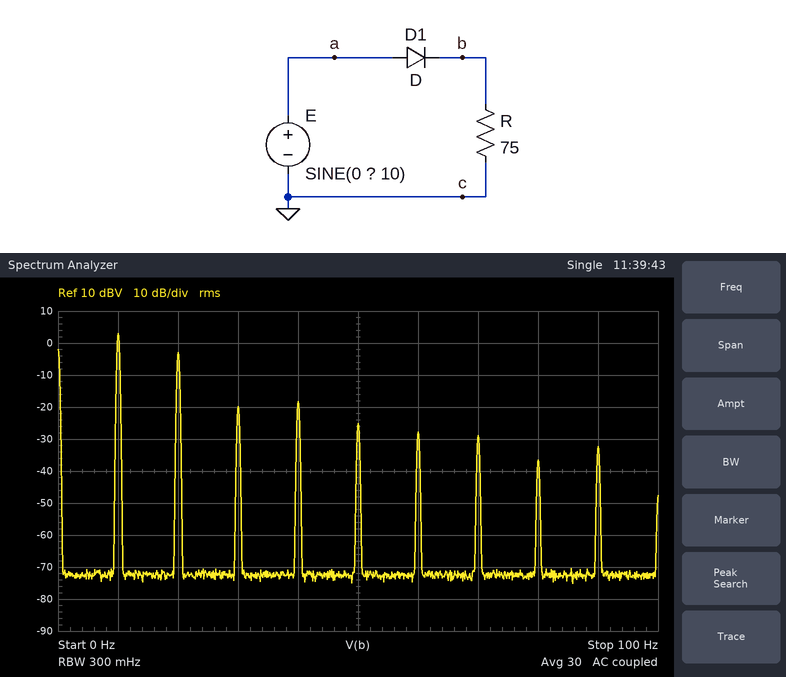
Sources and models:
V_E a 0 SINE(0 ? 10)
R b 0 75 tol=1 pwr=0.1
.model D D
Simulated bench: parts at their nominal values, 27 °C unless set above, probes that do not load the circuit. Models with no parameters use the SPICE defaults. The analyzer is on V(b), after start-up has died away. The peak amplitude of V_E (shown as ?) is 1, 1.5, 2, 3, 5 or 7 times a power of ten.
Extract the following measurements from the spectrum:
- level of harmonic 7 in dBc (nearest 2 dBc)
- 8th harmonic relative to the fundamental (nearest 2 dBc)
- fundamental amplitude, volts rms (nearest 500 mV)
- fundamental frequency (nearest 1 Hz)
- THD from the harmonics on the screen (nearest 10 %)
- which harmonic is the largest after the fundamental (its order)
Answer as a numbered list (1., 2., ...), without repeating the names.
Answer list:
1. -32 dBc
2. -40 dBc
3. 1.5 V
4. 10 Hz
5. 50 %
6. 2
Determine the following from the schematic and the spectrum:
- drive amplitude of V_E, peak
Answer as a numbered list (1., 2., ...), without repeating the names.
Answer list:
1. 5 V
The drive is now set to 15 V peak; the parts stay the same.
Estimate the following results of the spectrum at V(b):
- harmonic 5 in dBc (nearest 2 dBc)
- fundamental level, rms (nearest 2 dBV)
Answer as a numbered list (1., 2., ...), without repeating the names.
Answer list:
1. -38 dBc
2. 14 dBV
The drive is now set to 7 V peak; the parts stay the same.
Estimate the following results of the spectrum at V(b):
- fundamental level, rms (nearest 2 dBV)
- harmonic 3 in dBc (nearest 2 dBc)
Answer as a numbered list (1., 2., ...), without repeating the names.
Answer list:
1. 6 dBV
2. -26 dBc
